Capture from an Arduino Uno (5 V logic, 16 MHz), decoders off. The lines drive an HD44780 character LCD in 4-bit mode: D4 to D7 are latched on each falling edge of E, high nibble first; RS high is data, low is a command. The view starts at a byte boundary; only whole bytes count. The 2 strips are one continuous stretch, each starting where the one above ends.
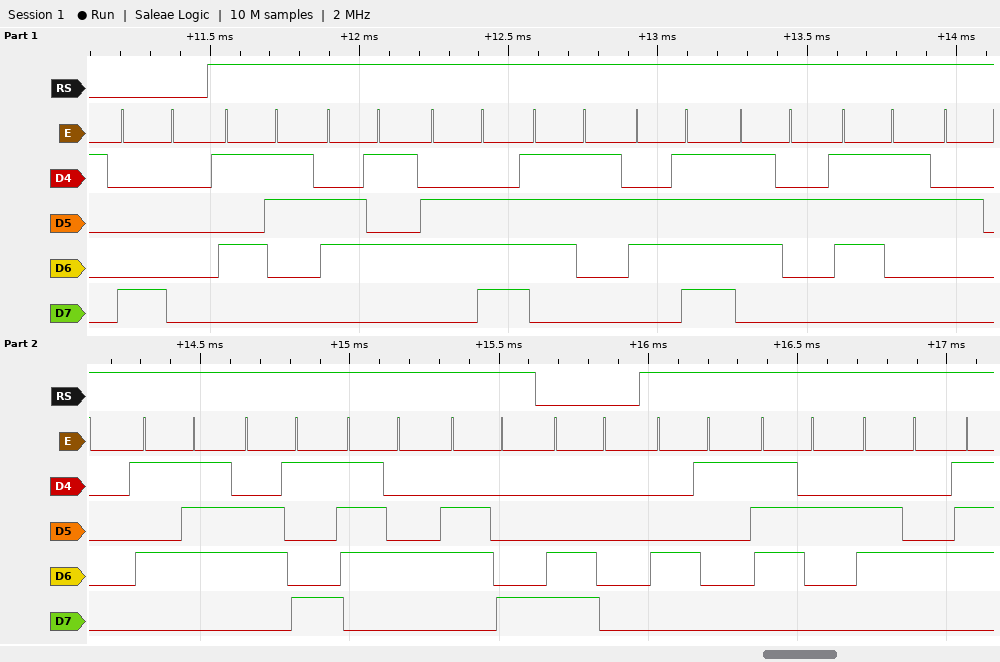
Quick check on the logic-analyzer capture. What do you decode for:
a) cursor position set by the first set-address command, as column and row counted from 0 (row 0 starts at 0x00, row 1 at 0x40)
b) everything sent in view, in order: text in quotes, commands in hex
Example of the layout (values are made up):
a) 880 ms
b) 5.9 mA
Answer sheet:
a) column 0, row 0
b) 0x80 "Sensors With" 0xC0 "Ard"
